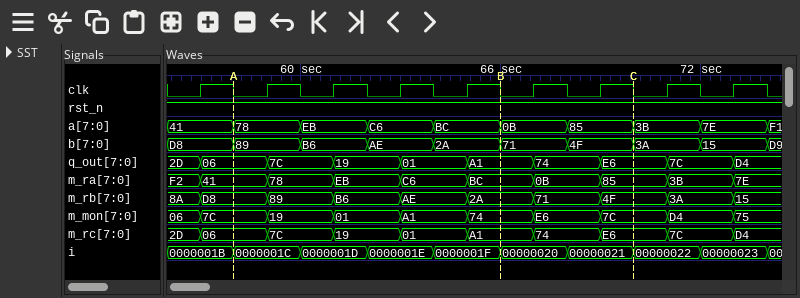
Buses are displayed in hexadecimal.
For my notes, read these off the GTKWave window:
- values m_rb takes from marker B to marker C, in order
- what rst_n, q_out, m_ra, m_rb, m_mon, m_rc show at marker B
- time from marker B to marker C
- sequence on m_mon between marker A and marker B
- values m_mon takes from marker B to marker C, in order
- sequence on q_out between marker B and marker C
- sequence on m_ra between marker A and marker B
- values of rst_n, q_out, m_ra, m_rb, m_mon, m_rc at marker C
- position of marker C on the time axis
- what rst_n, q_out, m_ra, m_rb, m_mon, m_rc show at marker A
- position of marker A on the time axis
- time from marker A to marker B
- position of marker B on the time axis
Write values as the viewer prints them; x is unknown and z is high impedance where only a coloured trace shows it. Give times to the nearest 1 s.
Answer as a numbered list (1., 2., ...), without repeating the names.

1. 2A, 71, 4F
2. rst_n=1, q_out=A1, m_ra=BC, m_rb=2A, m_mon=74, m_rc=A1
3. 4 s
4. 7C, 19, 01, A1, 74
5. 74, E6, 7C
6. A1, 74, E6
7. 41, 78, EB, C6, BC
8. rst_n=1, q_out=E6, m_ra=85, m_rb=4F, m_mon=7C, m_rc=E6
9. 70 s
10. rst_n=1, q_out=06, m_ra=41, m_rb=D8, m_mon=7C, m_rc=06
11. 58 s
12. 8 s
13. 66 s
